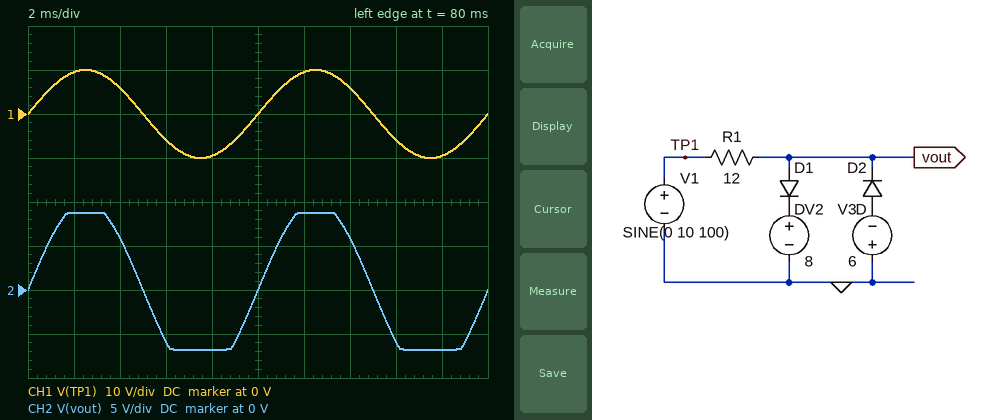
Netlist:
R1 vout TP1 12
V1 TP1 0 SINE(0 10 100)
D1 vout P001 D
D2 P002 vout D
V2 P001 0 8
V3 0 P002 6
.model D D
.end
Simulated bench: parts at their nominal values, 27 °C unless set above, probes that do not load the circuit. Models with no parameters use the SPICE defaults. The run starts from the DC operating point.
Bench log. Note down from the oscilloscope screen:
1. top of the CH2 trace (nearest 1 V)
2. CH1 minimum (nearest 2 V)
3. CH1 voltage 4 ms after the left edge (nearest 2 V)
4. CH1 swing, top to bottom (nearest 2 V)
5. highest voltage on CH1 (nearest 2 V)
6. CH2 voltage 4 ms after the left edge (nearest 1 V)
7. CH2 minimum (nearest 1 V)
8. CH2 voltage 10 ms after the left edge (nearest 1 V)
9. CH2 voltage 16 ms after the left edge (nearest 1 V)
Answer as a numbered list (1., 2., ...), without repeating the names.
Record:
1. 9 V
2. -10 V
3. 6 V
4. 20 V
5. 10 V
6. 6 V
7. -7 V
8. 0 V
9. -6 V
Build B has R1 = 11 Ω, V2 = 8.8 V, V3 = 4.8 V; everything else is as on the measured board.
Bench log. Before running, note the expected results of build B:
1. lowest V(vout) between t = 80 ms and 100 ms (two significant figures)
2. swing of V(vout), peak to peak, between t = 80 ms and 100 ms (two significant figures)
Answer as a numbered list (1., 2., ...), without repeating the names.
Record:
1. -5.6 V
2. 15 V
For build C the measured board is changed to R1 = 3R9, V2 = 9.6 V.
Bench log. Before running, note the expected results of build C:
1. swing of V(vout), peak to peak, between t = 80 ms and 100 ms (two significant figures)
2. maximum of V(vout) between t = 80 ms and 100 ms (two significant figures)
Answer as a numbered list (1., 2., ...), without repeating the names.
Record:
1. 17 V
2. 10 V
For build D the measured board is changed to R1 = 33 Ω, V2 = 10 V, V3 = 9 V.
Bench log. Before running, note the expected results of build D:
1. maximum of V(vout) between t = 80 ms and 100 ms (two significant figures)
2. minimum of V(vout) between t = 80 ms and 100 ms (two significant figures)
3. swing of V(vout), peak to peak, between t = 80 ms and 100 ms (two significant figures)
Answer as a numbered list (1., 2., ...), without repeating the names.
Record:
1. 10 V
2. -9.7 V
3. 20 V
